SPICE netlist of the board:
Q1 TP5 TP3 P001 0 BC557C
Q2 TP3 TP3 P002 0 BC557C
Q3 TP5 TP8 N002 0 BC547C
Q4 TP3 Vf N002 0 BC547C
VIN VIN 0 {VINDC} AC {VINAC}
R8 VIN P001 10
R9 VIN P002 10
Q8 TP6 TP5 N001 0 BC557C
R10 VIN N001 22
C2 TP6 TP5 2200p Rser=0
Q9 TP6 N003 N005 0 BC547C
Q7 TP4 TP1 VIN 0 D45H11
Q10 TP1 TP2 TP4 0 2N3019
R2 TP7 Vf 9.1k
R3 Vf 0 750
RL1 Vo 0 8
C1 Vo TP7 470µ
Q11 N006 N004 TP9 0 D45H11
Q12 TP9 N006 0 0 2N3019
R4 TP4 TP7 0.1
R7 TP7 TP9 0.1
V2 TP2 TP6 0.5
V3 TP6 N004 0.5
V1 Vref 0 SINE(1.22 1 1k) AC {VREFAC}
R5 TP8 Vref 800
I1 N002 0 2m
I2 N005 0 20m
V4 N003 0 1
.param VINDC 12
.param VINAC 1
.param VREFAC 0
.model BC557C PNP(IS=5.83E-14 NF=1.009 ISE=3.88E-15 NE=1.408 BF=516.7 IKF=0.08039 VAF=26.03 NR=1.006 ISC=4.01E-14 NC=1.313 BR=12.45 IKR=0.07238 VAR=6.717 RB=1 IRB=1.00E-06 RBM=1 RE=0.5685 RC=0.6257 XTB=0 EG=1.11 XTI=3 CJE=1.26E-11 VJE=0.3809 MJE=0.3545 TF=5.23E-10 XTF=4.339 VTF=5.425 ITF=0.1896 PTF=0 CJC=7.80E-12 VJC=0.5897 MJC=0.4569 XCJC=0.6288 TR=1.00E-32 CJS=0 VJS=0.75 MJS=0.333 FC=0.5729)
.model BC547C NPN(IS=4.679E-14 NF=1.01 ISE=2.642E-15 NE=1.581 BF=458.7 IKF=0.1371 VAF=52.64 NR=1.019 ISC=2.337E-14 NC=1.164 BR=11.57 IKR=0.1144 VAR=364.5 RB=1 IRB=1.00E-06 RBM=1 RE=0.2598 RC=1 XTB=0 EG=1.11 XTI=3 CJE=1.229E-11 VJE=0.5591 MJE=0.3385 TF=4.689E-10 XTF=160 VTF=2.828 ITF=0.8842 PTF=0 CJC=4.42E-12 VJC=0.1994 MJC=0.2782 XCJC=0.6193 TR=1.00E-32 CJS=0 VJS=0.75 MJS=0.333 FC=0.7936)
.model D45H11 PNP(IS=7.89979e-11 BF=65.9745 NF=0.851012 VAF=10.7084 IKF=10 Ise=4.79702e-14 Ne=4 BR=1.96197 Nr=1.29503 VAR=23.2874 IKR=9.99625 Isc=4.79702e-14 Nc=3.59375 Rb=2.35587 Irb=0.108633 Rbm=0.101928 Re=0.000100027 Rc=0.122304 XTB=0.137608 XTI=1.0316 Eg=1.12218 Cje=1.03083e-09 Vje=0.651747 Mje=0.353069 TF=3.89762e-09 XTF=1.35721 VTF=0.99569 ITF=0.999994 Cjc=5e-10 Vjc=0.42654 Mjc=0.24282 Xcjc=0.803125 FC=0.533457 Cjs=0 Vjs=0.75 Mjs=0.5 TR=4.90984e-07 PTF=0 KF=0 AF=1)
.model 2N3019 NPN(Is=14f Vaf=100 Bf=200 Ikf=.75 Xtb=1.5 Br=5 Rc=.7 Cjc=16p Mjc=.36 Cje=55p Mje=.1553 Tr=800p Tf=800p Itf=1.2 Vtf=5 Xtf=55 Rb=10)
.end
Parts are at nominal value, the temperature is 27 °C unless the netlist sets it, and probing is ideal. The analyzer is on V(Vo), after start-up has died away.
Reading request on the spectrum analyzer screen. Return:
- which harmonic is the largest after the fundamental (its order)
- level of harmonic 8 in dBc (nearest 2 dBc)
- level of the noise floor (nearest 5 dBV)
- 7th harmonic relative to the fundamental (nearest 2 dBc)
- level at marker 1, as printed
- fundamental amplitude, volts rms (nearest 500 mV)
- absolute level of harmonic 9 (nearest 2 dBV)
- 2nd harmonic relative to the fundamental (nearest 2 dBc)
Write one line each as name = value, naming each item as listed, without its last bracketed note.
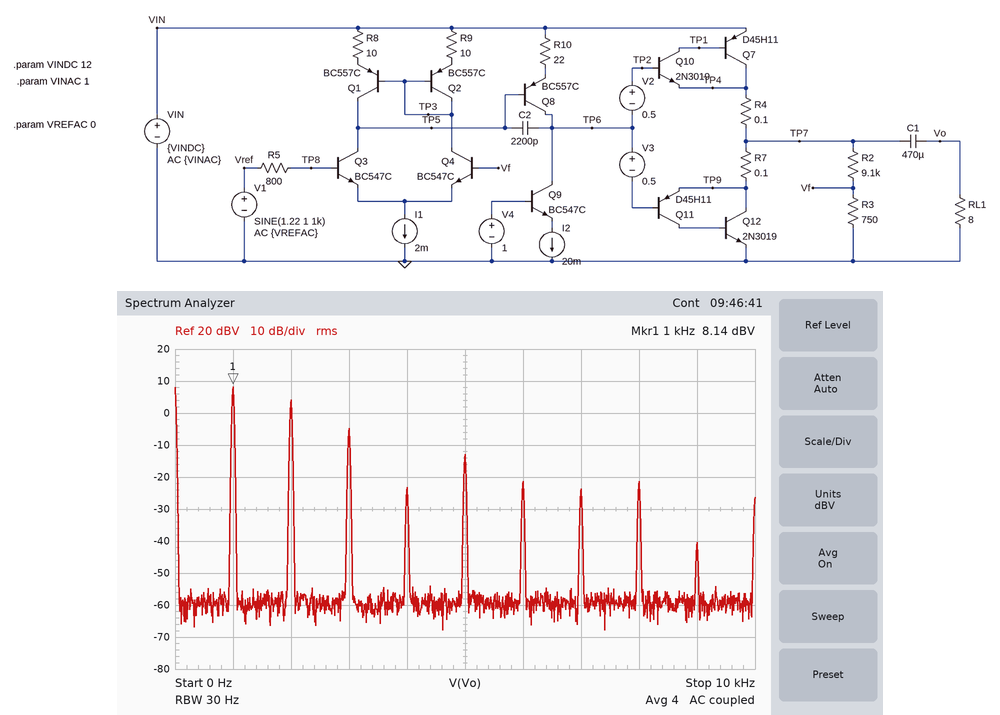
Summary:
which harmonic is the largest after the fundamental = 2
level of harmonic 8 in dBc = -30 dBc
level of the noise floor = -60 dBV
7th harmonic relative to the fundamental = -32 dBc
level at marker 1, as printed = 8.14 dBV
fundamental amplitude, volts rms = 2.5 V
absolute level of harmonic 9 = -40 dBV
2nd harmonic relative to the fundamental = -4 dBc
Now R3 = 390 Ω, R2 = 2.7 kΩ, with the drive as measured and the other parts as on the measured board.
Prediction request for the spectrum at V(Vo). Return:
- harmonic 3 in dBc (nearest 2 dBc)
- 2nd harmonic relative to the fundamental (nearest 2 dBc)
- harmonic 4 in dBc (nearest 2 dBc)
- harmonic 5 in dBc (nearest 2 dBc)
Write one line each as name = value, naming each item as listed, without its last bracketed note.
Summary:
harmonic 3 in dBc = -24 dBc
2nd harmonic relative to the fundamental = -10 dBc
harmonic 4 in dBc = -26 dBc
harmonic 5 in dBc = -30 dBc
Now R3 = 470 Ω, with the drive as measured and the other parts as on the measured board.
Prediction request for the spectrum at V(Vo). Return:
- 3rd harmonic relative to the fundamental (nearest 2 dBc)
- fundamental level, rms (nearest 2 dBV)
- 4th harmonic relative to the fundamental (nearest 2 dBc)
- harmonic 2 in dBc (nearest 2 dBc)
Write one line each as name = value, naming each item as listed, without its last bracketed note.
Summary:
3rd harmonic relative to the fundamental = -6 dBc
fundamental level, rms = 4 dBV
4th harmonic relative to the fundamental = -12 dBc
harmonic 2 in dBc = -2 dBc
